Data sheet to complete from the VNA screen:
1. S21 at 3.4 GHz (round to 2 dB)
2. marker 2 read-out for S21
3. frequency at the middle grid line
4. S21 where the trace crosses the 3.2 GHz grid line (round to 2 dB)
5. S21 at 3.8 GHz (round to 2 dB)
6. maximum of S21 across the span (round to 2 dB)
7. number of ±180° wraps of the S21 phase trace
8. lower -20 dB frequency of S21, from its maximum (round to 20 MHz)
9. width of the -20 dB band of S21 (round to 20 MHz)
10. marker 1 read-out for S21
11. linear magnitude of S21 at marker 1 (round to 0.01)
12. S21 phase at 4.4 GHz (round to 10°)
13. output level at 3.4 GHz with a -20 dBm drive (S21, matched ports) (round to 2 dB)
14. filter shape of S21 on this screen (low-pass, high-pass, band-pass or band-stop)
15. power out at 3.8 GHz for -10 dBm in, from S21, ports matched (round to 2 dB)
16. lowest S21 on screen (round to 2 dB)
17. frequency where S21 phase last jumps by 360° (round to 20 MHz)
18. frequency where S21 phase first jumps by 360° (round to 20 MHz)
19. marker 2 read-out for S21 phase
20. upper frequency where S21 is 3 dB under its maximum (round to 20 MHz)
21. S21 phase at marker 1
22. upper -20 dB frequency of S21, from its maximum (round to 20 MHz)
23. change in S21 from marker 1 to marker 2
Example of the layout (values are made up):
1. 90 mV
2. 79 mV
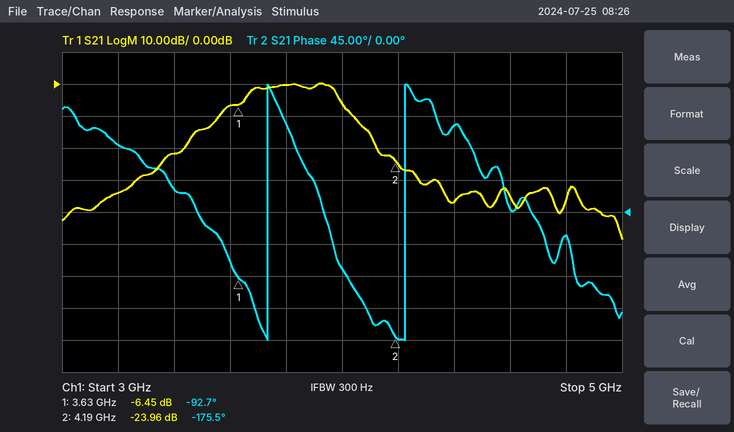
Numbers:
1. -22 dB
2. -23.96 dB
3. 4 GHz
4. -34 dB
5. 0 dB
6. 0 dB
7. 2
8. 3.44 GHz
9. 680 MHz
10. -6.45 dB
11. 0.48
12. 120°
13. -42 dBm
14. band-pass
15. -10 dBm
16. -48 dB
17. 4.22 GHz
18. 3.74 GHz
19. -175.5°
20. 3.98 GHz
21. -92.7°
22. 4.12 GHz
23. -17.51 dB
